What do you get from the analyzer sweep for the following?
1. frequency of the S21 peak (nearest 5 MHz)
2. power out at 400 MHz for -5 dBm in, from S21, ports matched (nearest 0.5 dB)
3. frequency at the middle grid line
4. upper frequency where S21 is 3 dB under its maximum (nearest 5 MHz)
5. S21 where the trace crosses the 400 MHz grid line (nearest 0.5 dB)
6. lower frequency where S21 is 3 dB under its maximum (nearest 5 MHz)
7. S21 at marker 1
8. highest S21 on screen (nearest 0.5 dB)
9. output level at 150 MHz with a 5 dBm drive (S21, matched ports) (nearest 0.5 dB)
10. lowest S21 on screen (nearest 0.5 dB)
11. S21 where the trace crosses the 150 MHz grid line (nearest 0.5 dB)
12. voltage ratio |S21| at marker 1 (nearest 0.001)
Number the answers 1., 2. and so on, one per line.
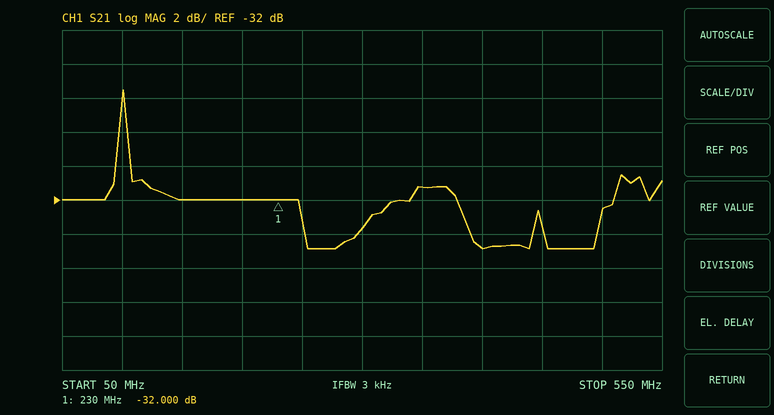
1. 100 MHz
2. -40.0 dBm
3. 300 MHz
4. 105 MHz
5. -35.0 dB
6. 95 MHz
7. -32.000 dB
8. -25.5 dB
9. -27.0 dBm
10. -35.0 dB
11. -32.0 dB
12. 0.025
